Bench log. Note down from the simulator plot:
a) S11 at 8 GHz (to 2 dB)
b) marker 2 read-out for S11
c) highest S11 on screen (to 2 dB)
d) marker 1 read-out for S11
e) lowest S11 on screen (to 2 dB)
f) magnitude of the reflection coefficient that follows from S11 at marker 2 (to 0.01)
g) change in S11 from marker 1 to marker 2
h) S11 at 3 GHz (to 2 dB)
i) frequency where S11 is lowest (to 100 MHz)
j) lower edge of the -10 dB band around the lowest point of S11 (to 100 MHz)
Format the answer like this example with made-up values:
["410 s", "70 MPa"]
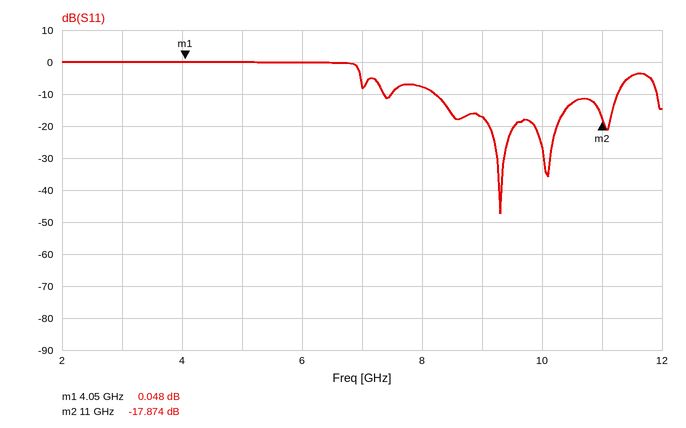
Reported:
["-8 dB", "-17.874 dB", "0 dB", "0.048 dB", "-48 dB", "0.13", "-17.922 dB", "0 dB", "9.3 GHz", "8.2 GHz"]
